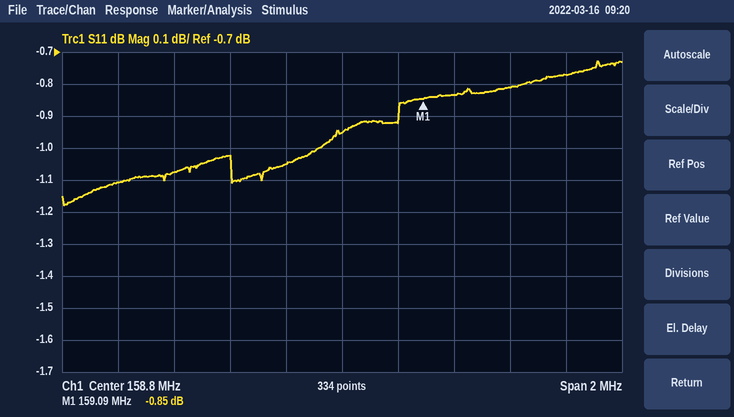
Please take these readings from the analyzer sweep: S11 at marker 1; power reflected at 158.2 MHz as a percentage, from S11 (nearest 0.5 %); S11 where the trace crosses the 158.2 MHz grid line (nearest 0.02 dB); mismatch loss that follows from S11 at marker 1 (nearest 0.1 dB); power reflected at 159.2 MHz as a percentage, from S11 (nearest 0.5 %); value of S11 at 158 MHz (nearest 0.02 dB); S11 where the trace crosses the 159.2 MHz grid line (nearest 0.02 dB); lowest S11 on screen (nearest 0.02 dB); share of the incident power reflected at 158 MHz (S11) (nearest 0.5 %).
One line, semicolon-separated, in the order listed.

-0.85 dB; 78.0 %; -1.08 dB; 7.5 dB; 82.5 %; -1.10 dB; -0.84 dB; -1.18 dB; 77.5 %
